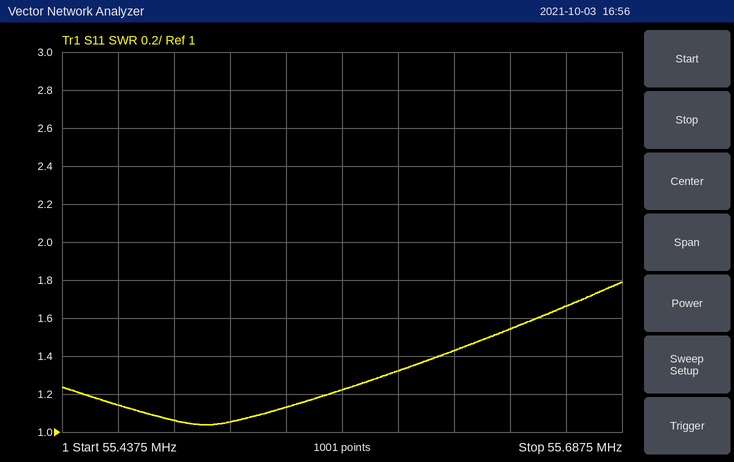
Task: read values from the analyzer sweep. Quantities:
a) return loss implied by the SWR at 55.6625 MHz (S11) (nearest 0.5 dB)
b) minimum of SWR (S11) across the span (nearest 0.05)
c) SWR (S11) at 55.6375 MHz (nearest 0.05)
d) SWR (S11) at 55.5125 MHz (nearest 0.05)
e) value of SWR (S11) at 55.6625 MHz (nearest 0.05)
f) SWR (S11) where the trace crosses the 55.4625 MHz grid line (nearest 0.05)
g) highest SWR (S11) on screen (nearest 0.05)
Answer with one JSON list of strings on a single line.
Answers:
["12.0 dB", "1.05", "1.55", "1.05", "1.65", "1.15", "1.80"]
